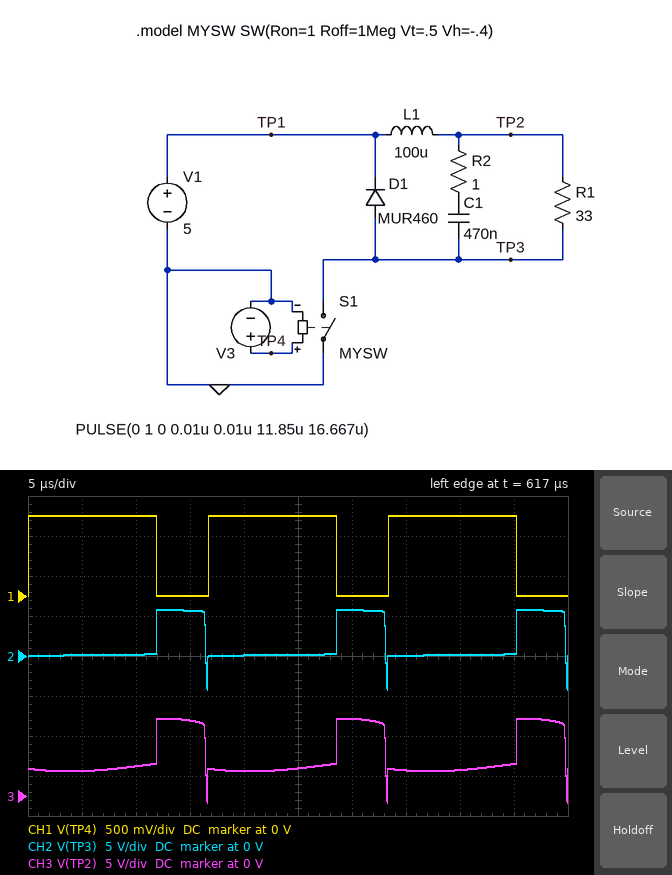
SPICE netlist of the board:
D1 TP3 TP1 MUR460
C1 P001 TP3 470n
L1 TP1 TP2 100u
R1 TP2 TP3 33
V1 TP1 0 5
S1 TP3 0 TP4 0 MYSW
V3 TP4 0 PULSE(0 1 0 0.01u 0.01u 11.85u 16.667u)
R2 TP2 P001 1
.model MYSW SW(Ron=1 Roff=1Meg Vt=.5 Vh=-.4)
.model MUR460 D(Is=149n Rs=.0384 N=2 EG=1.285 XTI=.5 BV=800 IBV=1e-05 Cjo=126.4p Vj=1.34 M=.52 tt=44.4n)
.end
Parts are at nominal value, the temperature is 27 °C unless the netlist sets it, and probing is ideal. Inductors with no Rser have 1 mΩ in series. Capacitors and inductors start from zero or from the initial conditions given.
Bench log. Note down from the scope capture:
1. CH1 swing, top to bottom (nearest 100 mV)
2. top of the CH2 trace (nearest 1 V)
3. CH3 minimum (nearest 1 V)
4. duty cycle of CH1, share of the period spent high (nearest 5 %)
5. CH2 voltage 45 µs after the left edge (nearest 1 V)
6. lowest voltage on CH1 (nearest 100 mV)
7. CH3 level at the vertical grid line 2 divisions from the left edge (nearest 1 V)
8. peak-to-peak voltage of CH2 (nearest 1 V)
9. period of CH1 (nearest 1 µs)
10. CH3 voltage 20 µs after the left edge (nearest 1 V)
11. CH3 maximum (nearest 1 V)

1.0 V
6 V
-1 V
70 %
0 V
0 V
4 V
10 V
17 µs
3 V
10 V
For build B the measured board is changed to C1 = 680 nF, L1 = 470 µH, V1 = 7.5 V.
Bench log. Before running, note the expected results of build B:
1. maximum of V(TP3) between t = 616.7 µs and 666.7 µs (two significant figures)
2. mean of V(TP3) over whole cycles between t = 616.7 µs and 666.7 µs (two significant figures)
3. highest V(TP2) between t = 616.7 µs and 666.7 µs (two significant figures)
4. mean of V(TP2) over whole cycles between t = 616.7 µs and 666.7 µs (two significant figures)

8.2 V
2.5 V
13 V
7.5 V
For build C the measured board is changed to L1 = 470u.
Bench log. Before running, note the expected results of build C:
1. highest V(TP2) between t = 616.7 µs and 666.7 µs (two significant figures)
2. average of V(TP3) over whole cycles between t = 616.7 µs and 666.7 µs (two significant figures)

9.1 V
1.7 V
